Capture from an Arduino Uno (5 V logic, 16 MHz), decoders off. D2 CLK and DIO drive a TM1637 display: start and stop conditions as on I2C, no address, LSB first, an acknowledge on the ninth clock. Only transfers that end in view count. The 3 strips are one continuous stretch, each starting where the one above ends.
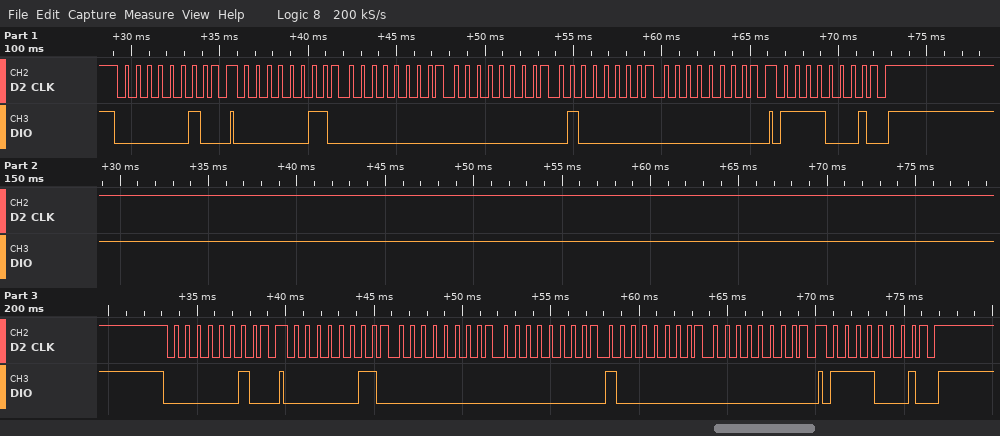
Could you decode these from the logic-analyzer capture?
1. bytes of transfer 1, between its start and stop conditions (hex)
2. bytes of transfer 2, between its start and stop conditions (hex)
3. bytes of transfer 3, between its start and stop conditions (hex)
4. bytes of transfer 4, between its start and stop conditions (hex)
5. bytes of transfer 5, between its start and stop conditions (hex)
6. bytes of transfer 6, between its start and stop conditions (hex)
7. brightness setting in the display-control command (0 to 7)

40
C0 00 00 02 00
8F
40
C0 00 00 01 00
8F
7
